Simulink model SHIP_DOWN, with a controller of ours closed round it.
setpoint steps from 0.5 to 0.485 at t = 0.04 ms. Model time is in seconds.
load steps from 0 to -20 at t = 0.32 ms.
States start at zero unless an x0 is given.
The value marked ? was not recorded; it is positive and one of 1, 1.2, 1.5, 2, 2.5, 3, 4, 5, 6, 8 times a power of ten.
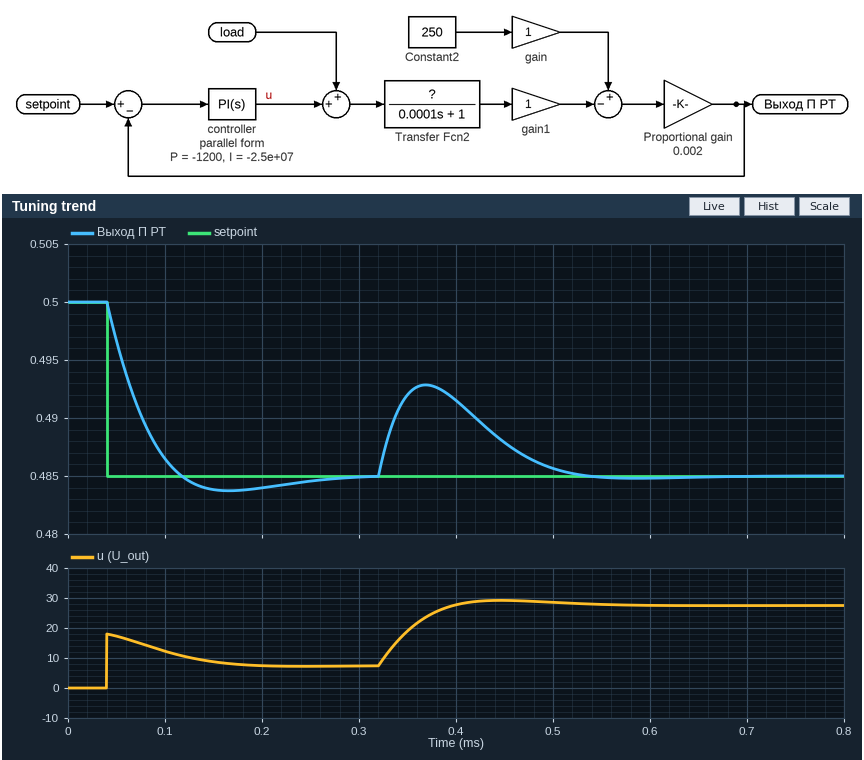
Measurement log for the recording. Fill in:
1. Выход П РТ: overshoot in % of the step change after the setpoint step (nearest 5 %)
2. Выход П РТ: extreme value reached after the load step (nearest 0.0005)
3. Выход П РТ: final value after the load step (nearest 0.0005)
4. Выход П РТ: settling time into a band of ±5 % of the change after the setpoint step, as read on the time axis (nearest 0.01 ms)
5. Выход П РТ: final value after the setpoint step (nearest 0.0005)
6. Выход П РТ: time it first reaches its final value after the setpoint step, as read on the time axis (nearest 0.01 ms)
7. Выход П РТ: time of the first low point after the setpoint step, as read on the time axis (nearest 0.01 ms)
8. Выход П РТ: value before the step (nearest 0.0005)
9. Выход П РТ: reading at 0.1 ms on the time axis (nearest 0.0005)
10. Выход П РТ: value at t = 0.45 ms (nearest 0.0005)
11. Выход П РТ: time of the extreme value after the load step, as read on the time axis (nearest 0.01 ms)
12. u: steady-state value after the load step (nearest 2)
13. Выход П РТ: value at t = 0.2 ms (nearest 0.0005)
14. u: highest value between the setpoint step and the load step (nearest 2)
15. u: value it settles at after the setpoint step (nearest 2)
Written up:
10 %
0.4930
0.4850
0.22 ms
0.4850
0.12 ms
0.17 ms
0.5000
0.4865
0.4880
0.37 ms
28
0.4840
18
8
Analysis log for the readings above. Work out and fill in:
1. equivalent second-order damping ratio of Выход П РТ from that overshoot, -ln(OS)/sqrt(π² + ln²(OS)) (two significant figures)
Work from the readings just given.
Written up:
0.59
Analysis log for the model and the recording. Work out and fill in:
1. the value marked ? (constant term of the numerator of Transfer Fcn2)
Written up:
1
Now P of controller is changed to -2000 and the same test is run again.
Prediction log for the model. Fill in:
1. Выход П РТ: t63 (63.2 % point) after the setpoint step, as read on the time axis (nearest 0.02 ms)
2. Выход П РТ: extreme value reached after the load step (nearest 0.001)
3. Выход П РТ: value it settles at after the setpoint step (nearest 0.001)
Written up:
0.06 ms
0.491
0.485
